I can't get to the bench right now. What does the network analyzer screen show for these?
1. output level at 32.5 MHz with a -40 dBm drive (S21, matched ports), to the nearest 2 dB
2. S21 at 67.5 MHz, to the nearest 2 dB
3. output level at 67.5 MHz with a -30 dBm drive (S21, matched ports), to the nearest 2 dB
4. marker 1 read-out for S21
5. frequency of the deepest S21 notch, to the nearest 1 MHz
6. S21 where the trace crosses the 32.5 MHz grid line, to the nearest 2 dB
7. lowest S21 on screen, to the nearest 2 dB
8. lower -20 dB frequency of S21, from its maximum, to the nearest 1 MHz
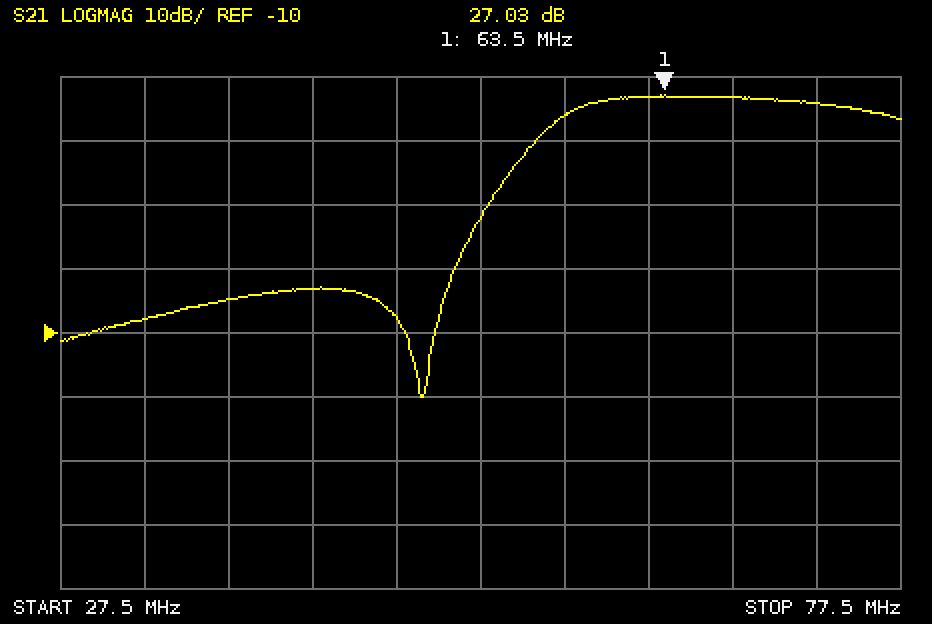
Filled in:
-48 dBm
26 dB
-4 dBm
27.03 dB
49 MHz
-8 dB
-20 dB
52 MHz
